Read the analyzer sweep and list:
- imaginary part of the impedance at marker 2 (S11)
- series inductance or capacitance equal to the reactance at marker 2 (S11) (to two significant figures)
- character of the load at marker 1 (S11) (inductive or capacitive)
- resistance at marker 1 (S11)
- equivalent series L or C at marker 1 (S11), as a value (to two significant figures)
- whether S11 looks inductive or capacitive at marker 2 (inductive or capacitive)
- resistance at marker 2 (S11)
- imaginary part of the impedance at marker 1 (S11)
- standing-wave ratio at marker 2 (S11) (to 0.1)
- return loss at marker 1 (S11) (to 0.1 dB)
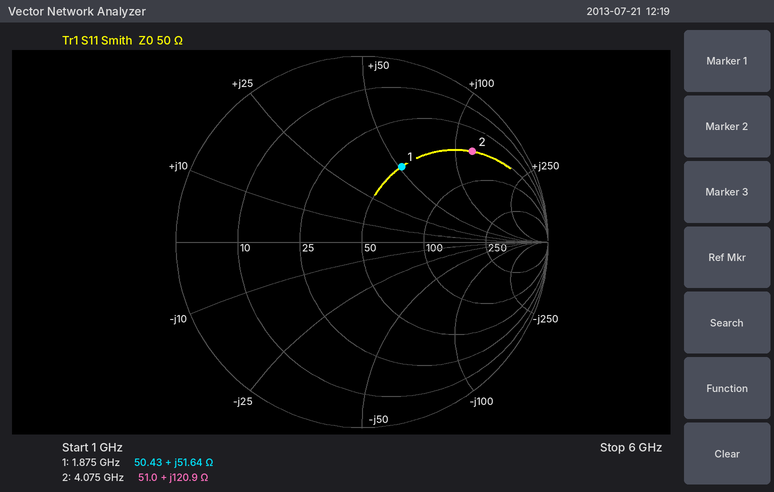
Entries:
+120.9 Ω
4.7 nH
inductive
50.43 Ω
4.4 nH
inductive
51.0 Ω
+51.64 Ω
7.6
6.8 dB
